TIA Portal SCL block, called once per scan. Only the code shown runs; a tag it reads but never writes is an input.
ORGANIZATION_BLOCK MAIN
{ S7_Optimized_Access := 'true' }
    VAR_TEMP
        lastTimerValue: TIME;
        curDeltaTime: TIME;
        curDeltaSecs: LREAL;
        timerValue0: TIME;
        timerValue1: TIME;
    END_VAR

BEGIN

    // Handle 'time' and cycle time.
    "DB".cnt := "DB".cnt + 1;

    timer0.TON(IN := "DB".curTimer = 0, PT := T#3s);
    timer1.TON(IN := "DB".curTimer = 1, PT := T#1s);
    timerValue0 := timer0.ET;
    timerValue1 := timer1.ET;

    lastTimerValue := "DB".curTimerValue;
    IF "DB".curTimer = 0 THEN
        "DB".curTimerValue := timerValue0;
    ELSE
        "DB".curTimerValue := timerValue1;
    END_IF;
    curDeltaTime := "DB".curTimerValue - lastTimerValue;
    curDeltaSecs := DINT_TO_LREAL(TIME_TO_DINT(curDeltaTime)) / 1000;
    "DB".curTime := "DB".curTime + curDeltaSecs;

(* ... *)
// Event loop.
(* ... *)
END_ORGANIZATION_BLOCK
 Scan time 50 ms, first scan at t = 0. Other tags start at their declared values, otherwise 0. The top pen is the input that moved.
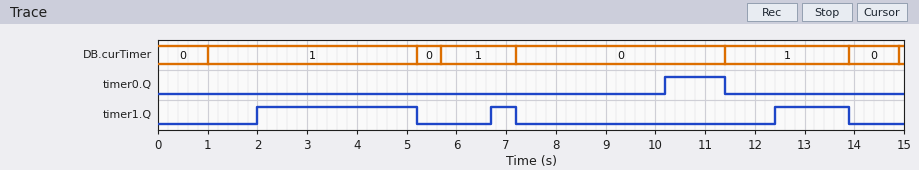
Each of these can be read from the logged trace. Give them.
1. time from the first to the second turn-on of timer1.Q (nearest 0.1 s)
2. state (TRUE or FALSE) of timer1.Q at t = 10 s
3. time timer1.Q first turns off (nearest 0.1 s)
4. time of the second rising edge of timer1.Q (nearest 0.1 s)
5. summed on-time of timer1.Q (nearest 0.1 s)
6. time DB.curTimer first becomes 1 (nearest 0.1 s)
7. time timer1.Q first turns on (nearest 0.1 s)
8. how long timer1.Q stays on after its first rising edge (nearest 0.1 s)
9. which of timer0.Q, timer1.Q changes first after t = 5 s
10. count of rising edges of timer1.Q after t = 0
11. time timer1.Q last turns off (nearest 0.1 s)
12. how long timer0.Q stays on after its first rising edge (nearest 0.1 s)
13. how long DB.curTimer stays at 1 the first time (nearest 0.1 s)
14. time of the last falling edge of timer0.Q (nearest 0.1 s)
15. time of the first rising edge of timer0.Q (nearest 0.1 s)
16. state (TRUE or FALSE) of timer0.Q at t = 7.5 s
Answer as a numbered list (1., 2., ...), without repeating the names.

1. 4.7 s
2. FALSE
3. 5.2 s
4. 6.7 s
5. 5.2 s
6. 1.0 s
7. 2.0 s
8. 3.2 s
9. timer1.Q
10. 3
11. 13.9 s
12. 1.2 s
13. 4.2 s
14. 11.4 s
15. 10.2 s
16. FALSE
